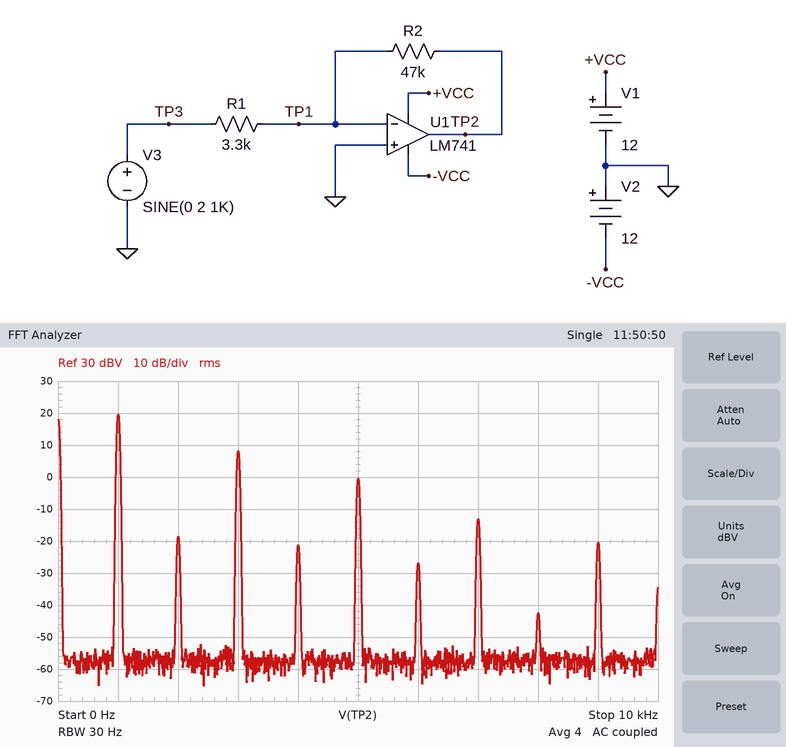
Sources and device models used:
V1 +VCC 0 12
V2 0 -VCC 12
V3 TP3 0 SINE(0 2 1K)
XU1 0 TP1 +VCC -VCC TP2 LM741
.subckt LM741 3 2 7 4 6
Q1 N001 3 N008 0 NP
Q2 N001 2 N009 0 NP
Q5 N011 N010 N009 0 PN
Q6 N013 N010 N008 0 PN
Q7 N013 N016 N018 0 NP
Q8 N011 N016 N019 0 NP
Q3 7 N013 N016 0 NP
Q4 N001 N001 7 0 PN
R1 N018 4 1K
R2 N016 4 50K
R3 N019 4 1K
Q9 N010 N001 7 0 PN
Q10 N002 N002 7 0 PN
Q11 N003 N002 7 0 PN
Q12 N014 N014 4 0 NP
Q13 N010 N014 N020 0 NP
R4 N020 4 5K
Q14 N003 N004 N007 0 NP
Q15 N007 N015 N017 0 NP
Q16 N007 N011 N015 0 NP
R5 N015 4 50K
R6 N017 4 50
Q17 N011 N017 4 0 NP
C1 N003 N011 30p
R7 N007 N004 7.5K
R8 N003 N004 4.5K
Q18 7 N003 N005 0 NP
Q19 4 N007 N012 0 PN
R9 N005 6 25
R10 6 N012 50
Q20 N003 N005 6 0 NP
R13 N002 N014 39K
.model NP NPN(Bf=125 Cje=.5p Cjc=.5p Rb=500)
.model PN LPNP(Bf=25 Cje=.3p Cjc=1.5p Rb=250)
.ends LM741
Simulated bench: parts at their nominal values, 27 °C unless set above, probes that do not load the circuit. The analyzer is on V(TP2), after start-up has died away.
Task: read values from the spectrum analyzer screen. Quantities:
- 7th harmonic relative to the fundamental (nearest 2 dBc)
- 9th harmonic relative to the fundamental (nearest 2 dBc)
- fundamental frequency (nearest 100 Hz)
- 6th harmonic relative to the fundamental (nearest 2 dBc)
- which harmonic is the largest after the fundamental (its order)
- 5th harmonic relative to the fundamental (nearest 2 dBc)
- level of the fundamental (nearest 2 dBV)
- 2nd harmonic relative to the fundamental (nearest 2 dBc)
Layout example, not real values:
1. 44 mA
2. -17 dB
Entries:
1. -32 dBc
2. -40 dBc
3. 1.0 kHz
4. -46 dBc
5. 3
6. -20 dBc
7. 20 dBV
8. -38 dBc
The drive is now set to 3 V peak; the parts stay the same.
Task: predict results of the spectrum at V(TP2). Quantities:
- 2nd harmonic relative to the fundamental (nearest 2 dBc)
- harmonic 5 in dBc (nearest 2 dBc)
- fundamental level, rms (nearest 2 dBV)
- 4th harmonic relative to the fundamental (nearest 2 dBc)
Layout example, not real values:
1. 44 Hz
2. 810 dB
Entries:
1. -42 dBc
2. -16 dBc
3. 20 dBV
4. -42 dBc
